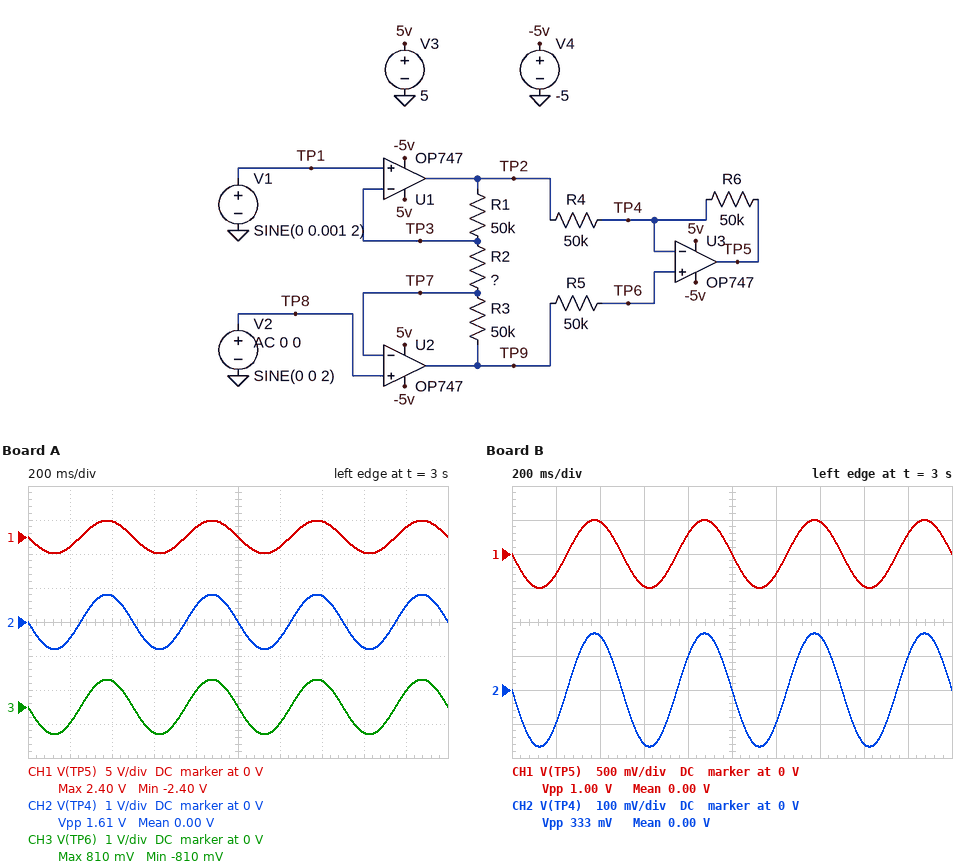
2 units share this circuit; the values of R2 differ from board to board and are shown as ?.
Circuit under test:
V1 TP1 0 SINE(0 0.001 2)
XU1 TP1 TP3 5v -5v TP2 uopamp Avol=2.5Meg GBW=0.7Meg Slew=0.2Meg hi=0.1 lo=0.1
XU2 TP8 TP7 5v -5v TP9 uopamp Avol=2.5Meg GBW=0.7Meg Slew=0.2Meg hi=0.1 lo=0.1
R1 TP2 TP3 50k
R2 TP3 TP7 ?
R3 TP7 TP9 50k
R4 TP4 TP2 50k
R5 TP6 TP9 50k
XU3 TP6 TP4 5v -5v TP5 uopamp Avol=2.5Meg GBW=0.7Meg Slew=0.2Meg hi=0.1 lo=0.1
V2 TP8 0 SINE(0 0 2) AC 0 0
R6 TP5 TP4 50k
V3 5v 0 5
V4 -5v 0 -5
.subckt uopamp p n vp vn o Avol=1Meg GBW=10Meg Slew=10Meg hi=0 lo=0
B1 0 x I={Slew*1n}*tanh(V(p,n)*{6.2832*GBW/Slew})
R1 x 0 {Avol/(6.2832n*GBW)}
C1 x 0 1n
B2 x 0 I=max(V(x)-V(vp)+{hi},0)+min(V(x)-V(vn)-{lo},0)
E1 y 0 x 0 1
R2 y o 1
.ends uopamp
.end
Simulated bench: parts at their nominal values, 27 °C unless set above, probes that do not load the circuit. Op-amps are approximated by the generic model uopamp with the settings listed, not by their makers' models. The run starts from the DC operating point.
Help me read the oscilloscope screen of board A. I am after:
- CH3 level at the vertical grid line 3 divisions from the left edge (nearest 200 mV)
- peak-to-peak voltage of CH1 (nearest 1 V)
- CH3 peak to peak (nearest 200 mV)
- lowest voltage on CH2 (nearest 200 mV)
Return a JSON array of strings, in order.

["-800 mV", "5 V", "1.6 V", "-800 mV"]
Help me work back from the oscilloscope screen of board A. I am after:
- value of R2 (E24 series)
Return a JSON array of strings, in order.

["62 Ω"]
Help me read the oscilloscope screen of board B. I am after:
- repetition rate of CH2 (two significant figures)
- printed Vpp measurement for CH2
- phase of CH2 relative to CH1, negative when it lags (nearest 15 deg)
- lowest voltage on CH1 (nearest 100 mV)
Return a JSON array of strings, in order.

["2.0 Hz", "333 mV", "0 deg", "-500 mV"]
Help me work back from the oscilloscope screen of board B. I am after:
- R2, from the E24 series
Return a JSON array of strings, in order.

["300 Ω"]
